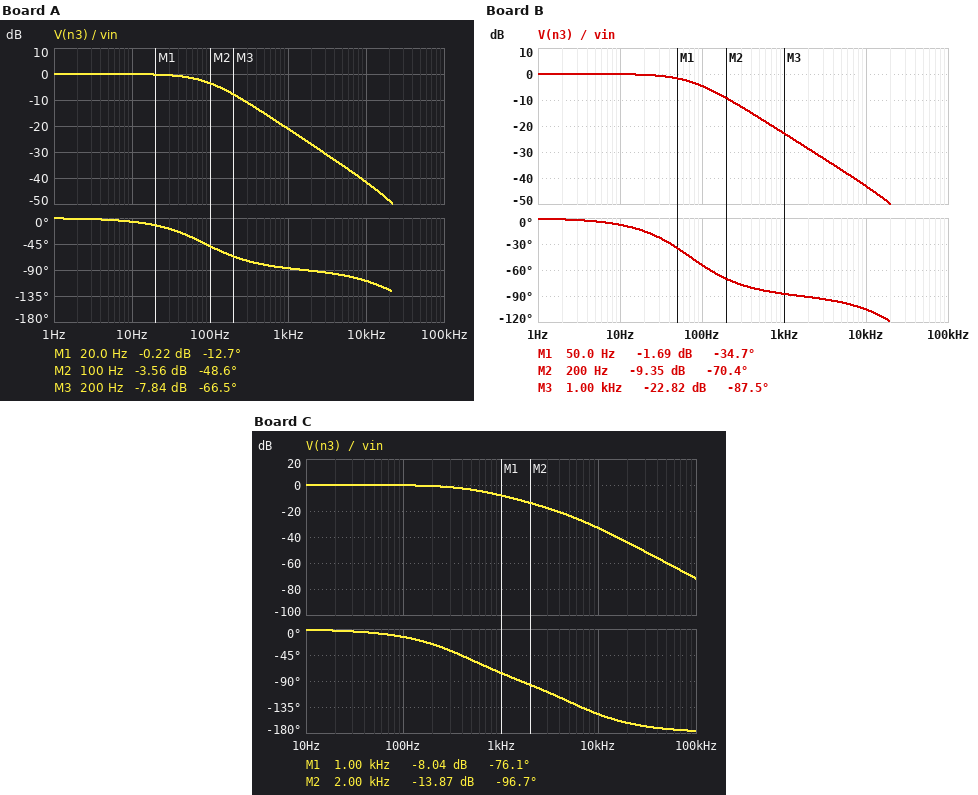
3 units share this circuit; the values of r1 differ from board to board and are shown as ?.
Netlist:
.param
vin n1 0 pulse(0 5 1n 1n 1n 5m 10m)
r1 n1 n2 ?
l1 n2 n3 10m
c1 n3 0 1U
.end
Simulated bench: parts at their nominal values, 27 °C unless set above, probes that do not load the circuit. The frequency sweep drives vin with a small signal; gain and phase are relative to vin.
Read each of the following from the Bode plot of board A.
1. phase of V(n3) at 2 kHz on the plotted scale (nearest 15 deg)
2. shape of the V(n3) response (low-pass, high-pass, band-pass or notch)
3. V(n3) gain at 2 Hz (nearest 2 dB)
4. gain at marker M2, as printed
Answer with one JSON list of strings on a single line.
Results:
["-90 deg", "low-pass", "0 dB", "-3.56 dB"]
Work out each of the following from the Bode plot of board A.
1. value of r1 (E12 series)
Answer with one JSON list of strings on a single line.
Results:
["1.8 kΩ"]
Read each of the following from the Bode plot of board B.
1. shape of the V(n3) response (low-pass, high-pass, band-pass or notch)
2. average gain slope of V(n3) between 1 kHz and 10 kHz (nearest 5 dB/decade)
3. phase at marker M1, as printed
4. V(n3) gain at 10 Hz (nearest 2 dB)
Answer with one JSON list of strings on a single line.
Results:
["low-pass", "-20 dB/decade", "-34.7 deg", "0 dB"]
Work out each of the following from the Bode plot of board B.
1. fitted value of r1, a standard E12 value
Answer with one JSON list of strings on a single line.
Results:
["2.2 kΩ"]
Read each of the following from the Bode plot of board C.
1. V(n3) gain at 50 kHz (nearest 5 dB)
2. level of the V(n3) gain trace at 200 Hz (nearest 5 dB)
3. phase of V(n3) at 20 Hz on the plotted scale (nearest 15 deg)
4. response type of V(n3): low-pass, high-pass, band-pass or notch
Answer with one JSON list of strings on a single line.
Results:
["-60 dB", "0 dB", "0 deg", "low-pass"]
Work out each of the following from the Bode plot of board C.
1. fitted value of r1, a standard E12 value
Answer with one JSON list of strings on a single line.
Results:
["390 Ω"]
